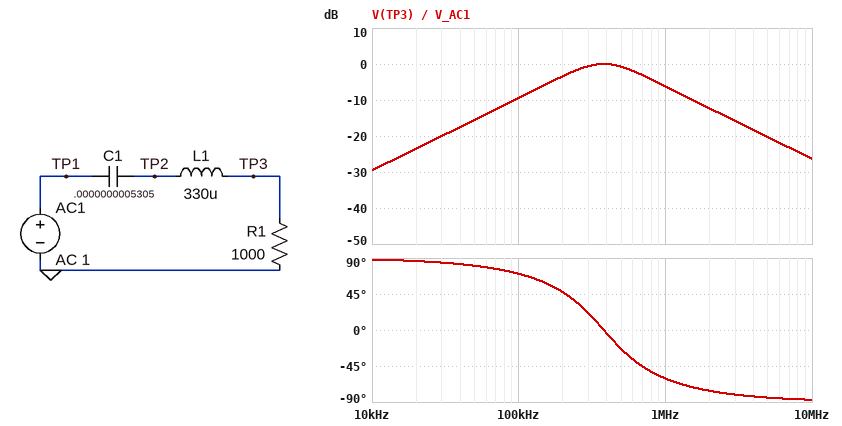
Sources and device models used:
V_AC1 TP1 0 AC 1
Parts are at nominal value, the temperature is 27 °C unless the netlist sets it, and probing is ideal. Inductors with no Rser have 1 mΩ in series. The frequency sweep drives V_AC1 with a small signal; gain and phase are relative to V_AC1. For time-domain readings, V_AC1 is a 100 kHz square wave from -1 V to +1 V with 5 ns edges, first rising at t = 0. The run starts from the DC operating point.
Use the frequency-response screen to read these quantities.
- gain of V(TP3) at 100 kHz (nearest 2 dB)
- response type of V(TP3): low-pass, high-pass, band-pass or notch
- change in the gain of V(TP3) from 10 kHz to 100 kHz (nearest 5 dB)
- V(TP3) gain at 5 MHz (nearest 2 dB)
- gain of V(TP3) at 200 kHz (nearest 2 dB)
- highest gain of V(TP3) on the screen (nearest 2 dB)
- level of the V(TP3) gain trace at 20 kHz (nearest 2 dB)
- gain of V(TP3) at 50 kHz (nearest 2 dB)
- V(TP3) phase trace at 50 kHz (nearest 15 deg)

-10 dB
band-pass
20 dB
-20 dB
-4 dB
0 dB
-24 dB
-16 dB
75 deg
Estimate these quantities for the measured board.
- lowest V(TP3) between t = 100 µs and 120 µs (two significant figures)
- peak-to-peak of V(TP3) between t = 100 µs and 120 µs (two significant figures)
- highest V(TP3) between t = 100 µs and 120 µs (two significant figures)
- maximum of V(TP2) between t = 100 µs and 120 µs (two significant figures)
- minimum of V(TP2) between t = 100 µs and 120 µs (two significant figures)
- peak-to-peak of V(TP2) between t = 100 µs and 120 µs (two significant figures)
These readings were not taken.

-1.2 V
2.5 V
1.2 V
2.0 V
-2.0 V
4.0 V
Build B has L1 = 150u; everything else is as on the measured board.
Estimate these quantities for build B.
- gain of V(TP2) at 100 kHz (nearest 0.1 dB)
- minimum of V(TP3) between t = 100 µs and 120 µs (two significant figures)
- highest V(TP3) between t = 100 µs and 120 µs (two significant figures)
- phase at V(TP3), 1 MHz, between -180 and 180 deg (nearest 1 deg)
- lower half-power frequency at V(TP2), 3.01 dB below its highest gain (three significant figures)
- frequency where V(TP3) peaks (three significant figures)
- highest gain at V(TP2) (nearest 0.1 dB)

-9.7 dB
-1.4 V
1.4 V
-33 deg
292 kHz
564 kHz
1.4 dB
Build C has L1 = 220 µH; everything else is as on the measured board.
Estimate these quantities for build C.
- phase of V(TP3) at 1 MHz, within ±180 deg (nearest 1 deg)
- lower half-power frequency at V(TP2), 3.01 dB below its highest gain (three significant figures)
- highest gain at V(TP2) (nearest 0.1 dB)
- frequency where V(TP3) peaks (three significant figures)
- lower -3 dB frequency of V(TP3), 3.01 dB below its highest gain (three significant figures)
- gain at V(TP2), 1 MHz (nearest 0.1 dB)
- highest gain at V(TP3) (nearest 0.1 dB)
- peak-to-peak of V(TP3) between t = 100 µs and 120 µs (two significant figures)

-47 deg
275 kHz
1.8 dB
466 kHz
228 kHz
1.3 dB
0 dB
2.7 V
